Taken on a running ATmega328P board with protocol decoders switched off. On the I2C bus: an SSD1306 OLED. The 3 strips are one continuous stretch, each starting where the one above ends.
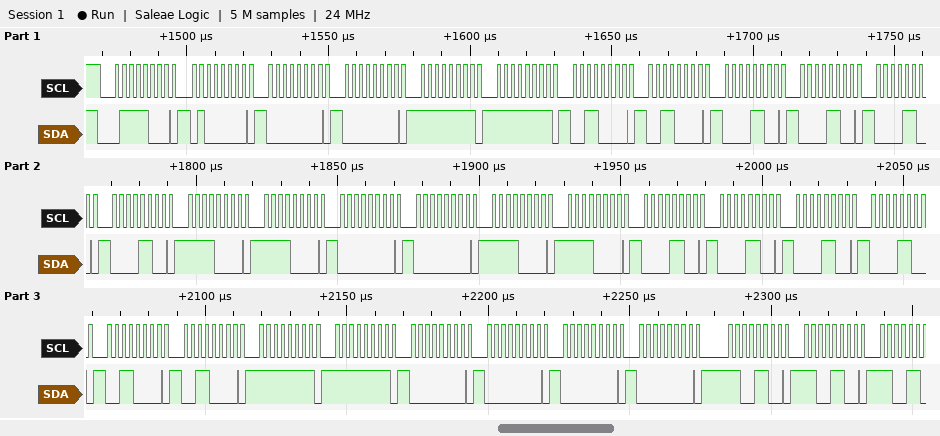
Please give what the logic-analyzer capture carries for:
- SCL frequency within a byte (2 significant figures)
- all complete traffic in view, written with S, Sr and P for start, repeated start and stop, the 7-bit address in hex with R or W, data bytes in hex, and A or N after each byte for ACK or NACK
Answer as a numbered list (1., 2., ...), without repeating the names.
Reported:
1. 400 kHz
2. S 3CW A 40 A 00 A 00 A FF A FF A 30 A 30 A 0C A 0C A 0C A 0C A F0 A F0 A 00 A 00 A F0 A F0 A 0C A 0C A 0C A 0C A 30 A 30 A FF A FF A 00 A 00 A 00 A 00 A CC A CC A
